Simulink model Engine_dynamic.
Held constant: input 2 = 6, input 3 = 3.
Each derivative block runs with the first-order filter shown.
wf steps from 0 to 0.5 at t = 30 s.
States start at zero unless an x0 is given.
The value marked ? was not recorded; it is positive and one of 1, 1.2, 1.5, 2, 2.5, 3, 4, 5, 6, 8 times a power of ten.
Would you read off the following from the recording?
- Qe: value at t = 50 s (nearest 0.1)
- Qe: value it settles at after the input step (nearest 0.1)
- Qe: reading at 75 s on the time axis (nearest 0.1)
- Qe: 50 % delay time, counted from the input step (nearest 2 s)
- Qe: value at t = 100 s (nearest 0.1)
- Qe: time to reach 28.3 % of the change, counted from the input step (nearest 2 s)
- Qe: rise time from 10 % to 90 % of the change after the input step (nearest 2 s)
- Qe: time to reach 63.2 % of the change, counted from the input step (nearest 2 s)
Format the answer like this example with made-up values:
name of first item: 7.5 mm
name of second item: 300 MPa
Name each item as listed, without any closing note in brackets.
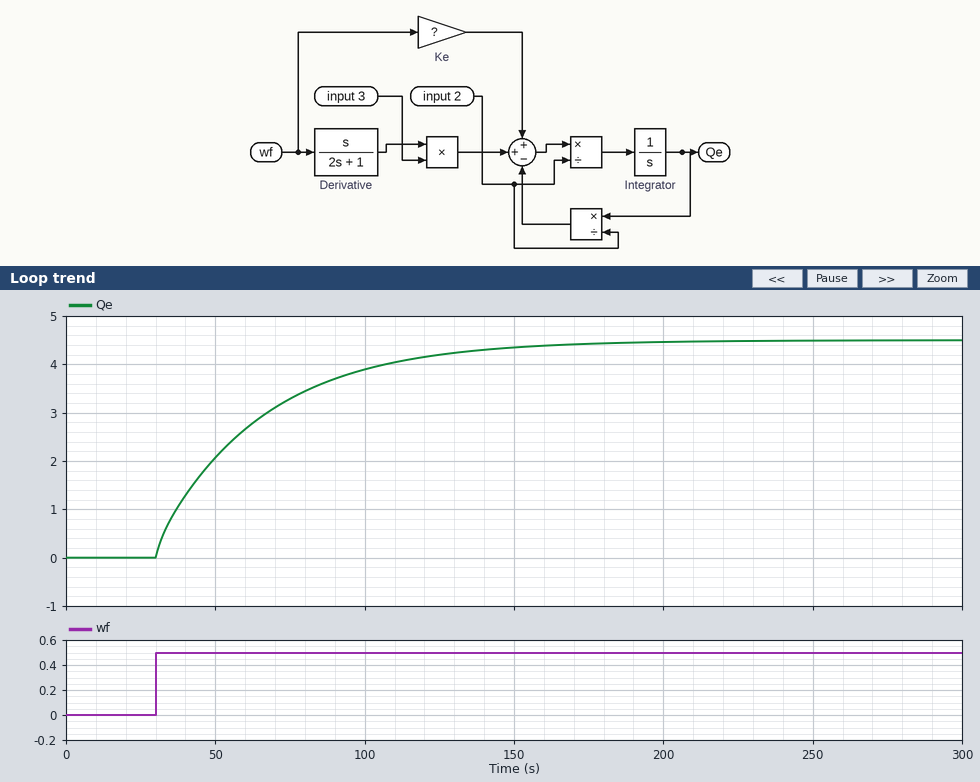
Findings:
Qe: value at t = 50 s: 2.1
Qe: value it settles at after the input step: 4.5
Qe: reading at 75 s on the time axis: 3.3
Qe: 50 % delay time, counted from the input step: 22 s
Qe: value at t = 100 s: 3.9
Qe: time to reach 28.3 % of the change, counted from the input step: 10 s
Qe: rise time from 10 % to 90 % of the change after the input step: 78 s
Qe: time to reach 63.2 % of the change, counted from the input step: 34 s
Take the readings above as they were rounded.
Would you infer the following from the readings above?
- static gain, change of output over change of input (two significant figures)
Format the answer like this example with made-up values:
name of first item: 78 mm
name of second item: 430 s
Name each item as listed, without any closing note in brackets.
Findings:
static gain, change of output over change of input: 9.0
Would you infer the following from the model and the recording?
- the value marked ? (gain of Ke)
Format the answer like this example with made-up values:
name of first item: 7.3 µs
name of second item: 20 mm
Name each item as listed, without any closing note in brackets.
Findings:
the value marked ?: 1.5
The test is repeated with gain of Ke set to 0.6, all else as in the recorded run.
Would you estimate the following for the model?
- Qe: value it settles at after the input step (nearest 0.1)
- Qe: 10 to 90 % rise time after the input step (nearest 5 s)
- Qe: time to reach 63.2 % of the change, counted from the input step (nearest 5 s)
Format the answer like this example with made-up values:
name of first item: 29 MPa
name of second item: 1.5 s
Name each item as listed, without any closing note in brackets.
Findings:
Qe: value it settles at after the input step: 1.8
Qe: 10 to 90 % rise time after the input step: 75 s
Qe: time to reach 63.2 % of the change, counted from the input step: 30 s
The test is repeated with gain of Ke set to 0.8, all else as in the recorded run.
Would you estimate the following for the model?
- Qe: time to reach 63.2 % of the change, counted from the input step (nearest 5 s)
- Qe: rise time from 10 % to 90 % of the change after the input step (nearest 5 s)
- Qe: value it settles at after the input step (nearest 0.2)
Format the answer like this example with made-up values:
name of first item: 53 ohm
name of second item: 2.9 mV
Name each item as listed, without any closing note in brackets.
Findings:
Qe: time to reach 63.2 % of the change, counted from the input step: 30 s
Qe: rise time from 10 % to 90 % of the change after the input step: 75 s
Qe: value it settles at after the input step: 2.4
